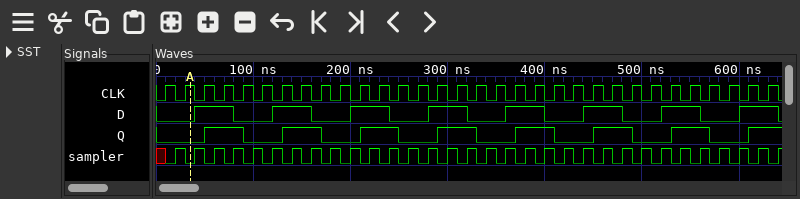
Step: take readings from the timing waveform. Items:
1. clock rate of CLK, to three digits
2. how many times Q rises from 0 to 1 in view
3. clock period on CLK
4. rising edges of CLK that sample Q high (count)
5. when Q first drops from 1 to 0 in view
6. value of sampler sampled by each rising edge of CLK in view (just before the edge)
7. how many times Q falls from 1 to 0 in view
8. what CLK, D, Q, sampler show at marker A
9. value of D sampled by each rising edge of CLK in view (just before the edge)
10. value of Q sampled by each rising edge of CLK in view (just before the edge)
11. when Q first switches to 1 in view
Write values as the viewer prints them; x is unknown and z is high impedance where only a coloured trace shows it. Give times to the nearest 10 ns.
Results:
50.0 MHz
8
20 ns
15
90 ns
x 1 1 1 1 1 1 1 1 1 1 1 1 1 1 1 1 1 1 1 1 1 1 1 1 1 1 1 1 1 1 1
7
CLK=1, D=0, Q=0, sampler=0
0 0 1 1 0 0 1 1 0 0 1 1 0 0 1 1 0 0 1 1 0 0 1 1 0 0 1 1 0 0 1 1
0 0 0 1 1 0 0 1 1 0 0 1 1 0 0 1 1 0 0 1 1 0 0 1 1 0 0 1 1 0 0 1
50 ns
